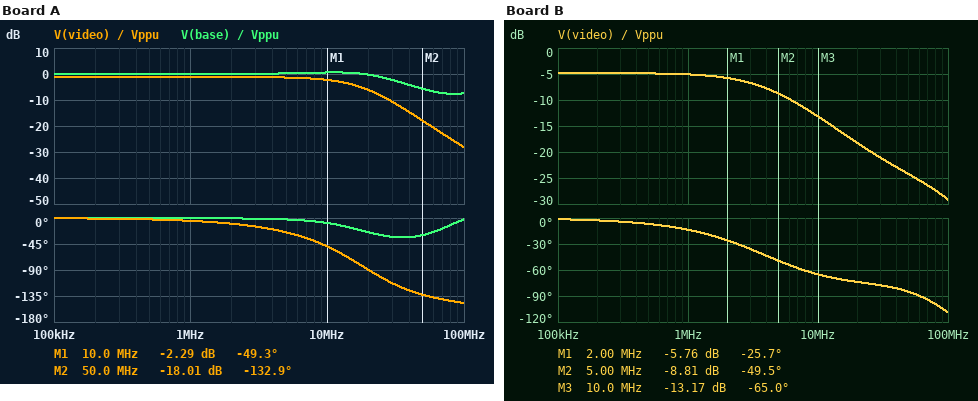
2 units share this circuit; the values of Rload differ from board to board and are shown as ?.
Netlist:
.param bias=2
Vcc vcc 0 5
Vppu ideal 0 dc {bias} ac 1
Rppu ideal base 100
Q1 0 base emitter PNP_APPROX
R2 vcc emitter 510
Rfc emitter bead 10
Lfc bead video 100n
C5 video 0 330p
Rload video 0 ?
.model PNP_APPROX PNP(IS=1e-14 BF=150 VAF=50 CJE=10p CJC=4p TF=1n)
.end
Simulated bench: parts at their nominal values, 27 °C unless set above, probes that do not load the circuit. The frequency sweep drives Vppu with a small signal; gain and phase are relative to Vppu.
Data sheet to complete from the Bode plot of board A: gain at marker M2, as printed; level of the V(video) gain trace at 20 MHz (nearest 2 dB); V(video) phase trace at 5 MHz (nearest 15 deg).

-18.01 dB
-6 dB
-30 deg
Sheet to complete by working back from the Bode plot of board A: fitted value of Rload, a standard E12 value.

680 Ω
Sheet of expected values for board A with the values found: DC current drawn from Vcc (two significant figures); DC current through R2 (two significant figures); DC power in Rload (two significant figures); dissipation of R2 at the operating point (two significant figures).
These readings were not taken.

4.6 mA
4.6 mA
10 mW
11 mW
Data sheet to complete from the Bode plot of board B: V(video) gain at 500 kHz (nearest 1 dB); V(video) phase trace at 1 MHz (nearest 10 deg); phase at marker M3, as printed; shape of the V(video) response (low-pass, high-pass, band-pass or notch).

-5 dB
-10 deg
-65.0 deg
low-pass
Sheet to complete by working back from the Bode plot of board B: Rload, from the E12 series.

560 Ω
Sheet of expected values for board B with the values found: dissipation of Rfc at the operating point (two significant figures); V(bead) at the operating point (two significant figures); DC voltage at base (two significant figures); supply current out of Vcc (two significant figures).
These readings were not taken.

210 µW
2.6 V
2.0 V
4.7 mA
